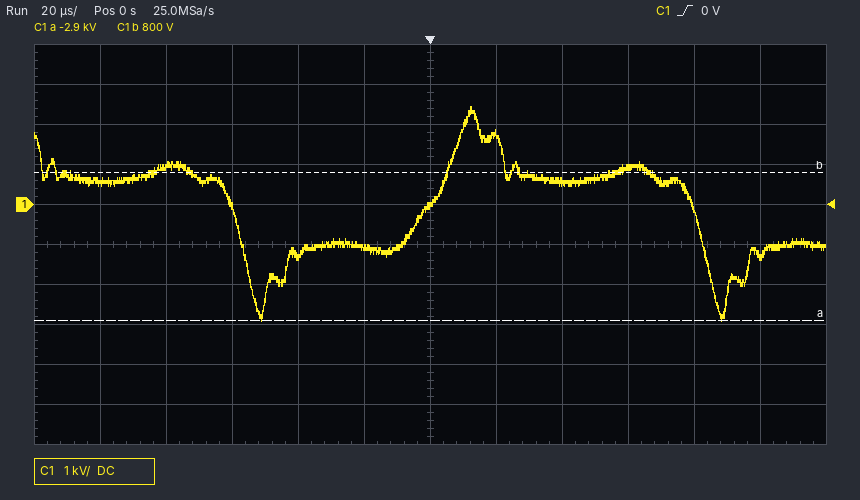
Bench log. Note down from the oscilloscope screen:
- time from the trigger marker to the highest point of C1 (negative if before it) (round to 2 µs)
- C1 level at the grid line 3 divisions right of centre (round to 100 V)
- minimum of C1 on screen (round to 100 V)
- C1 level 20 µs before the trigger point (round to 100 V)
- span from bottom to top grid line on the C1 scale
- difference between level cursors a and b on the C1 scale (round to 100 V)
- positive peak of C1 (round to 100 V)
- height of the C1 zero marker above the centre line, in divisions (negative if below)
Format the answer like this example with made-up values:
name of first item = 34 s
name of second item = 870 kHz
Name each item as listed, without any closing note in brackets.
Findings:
time from the trigger marker to the highest point of C1 (negative if before it) = +12 µs
C1 level at the grid line 3 divisions right of centre = 900 V
minimum of C1 on screen = -2.9 kV
C1 level 20 µs before the trigger point = -1.1 kV
span from bottom to top grid line on the C1 scale = 10 kV
difference between level cursors a and b on the C1 scale = 3.7 kV
positive peak of C1 = 2.4 kV
height of the C1 zero marker above the centre line, in divisions = +1.0 div
